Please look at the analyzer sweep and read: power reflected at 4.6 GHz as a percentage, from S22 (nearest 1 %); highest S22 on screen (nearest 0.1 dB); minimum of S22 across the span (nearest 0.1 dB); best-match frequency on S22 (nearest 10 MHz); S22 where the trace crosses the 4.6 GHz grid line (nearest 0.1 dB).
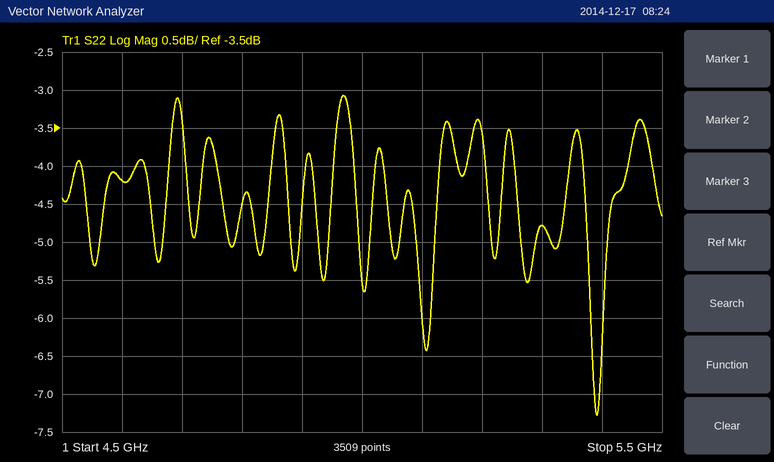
38 %
-3.1 dB
-7.3 dB
5.39 GHz
-4.2 dB
